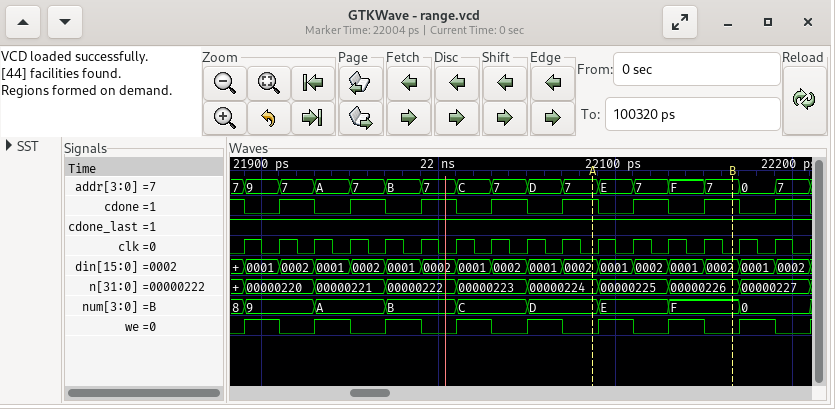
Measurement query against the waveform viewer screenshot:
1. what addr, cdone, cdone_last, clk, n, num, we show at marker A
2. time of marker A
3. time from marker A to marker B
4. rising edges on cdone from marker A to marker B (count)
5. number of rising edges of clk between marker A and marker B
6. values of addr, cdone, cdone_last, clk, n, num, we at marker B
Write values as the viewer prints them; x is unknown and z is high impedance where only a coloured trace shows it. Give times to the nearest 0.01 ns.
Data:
addr=7, cdone=1, cdone_last=1, clk=0, n=00000224, num=D, we=0
22.09 ns
0.08 ns
2
4
addr=7, cdone=1, cdone_last=1, clk=0, n=00000226, num=F, we=0
